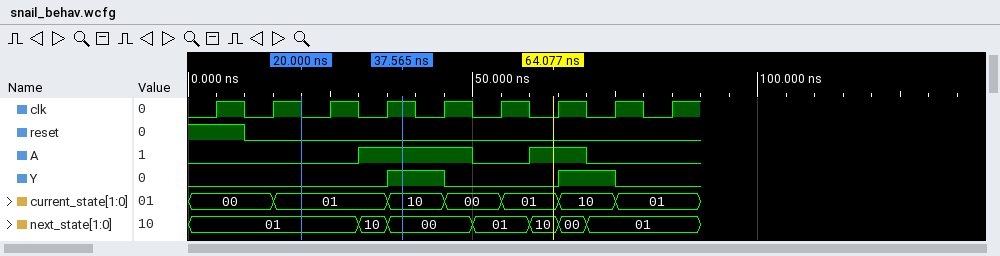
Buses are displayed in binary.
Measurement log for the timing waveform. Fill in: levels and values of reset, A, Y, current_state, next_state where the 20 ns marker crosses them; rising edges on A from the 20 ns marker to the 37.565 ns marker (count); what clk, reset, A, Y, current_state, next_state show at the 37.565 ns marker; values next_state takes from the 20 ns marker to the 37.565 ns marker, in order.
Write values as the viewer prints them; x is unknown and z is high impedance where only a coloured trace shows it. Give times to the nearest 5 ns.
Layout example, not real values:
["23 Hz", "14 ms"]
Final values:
["reset=0, A=0, Y=0, current_state=01, next_state=01", "1", "clk=1, reset=0, A=1, Y=1, current_state=10, next_state=00", "01, 10, 00"]
